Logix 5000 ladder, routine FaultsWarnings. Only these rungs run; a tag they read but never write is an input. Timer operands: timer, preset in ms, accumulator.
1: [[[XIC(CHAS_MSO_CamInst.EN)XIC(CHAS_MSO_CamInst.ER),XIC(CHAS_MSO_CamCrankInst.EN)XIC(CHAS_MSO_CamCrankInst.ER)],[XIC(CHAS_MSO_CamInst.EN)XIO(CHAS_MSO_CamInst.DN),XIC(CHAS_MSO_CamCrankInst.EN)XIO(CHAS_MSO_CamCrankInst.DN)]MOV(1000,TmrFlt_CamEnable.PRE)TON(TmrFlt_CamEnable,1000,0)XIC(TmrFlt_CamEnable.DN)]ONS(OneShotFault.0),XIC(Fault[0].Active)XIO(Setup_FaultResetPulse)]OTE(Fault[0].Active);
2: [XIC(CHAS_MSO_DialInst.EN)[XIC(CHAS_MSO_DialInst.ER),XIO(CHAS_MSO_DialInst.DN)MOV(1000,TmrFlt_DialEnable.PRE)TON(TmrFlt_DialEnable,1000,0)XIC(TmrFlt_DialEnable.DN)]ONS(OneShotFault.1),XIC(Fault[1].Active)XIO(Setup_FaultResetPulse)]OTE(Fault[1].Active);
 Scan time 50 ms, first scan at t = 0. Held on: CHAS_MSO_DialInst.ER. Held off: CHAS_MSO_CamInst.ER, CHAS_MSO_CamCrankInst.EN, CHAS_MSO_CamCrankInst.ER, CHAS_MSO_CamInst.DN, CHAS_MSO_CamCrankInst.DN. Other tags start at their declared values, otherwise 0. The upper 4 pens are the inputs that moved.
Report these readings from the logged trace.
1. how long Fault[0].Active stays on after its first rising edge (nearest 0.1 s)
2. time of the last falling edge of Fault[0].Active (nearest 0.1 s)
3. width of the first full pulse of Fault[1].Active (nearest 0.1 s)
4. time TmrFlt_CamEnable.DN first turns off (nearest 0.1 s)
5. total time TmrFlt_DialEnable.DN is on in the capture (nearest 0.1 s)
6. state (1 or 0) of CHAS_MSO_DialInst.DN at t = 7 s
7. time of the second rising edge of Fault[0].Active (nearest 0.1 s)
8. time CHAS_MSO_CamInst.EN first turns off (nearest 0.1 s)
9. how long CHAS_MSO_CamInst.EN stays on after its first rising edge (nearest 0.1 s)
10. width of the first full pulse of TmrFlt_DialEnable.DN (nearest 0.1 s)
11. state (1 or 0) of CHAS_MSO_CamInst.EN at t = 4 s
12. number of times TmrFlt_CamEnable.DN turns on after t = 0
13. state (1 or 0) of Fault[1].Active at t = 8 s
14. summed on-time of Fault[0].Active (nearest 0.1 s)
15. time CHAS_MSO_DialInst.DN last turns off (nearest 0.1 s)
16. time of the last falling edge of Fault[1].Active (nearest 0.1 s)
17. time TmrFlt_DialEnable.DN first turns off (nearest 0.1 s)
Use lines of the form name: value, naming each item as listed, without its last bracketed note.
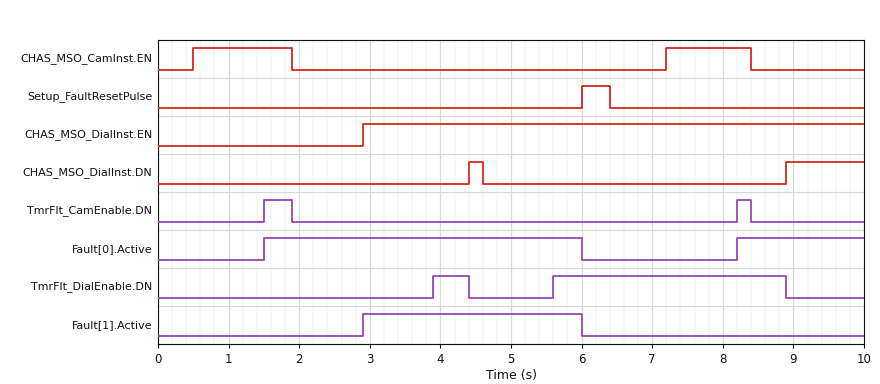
how long Fault[0].Active stays on after its first rising edge: 4.5 s
time of the last falling edge of Fault[0].Active: 6.0 s
width of the first full pulse of Fault[1].Active: 3.1 s
time TmrFlt_CamEnable.DN first turns off: 1.9 s
total time TmrFlt_DialEnable.DN is on in the capture: 3.8 s
state (1 or 0) of CHAS_MSO_DialInst.DN at t = 7 s: 0
time of the second rising edge of Fault[0].Active: 8.2 s
time CHAS_MSO_CamInst.EN first turns off: 1.9 s
how long CHAS_MSO_CamInst.EN stays on after its first rising edge: 1.4 s
width of the first full pulse of TmrFlt_DialEnable.DN: 0.5 s
state (1 or 0) of CHAS_MSO_CamInst.EN at t = 4 s: 0
number of times TmrFlt_CamEnable.DN turns on after t = 0: 2
state (1 or 0) of Fault[1].Active at t = 8 s: 0
summed on-time of Fault[0].Active: 6.3 s
time CHAS_MSO_DialInst.DN last turns off: 4.6 s
time of the last falling edge of Fault[1].Active: 6.0 s
time TmrFlt_DialEnable.DN first turns off: 4.4 s
